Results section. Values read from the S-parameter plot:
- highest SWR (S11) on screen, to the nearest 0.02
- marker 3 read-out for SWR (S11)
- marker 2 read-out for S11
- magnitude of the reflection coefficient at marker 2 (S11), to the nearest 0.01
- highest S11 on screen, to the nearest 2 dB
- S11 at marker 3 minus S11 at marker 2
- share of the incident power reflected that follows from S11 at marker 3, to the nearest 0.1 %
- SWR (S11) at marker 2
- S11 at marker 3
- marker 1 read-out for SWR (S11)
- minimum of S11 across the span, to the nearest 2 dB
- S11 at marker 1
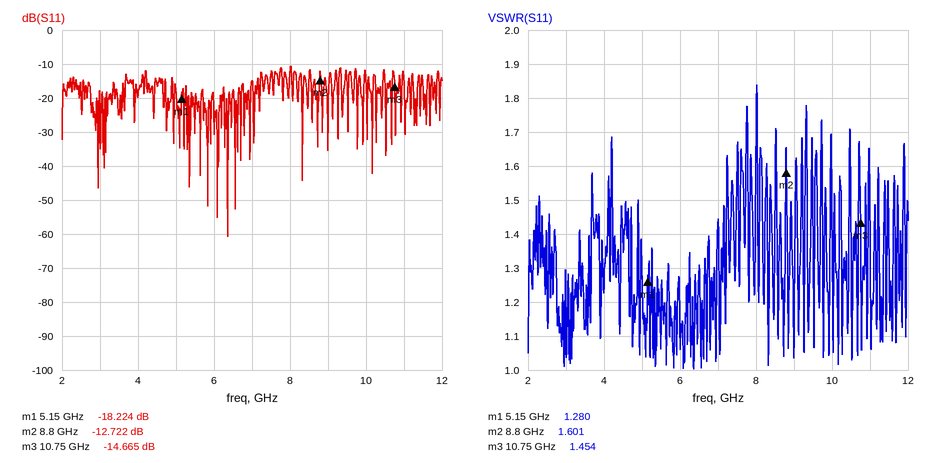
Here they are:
1.84
1.454
-12.722 dB
0.23
-10 dB
-1.943 dB
3.4 %
1.601
-14.665 dB
1.280
-60 dB
-18.224 dB
